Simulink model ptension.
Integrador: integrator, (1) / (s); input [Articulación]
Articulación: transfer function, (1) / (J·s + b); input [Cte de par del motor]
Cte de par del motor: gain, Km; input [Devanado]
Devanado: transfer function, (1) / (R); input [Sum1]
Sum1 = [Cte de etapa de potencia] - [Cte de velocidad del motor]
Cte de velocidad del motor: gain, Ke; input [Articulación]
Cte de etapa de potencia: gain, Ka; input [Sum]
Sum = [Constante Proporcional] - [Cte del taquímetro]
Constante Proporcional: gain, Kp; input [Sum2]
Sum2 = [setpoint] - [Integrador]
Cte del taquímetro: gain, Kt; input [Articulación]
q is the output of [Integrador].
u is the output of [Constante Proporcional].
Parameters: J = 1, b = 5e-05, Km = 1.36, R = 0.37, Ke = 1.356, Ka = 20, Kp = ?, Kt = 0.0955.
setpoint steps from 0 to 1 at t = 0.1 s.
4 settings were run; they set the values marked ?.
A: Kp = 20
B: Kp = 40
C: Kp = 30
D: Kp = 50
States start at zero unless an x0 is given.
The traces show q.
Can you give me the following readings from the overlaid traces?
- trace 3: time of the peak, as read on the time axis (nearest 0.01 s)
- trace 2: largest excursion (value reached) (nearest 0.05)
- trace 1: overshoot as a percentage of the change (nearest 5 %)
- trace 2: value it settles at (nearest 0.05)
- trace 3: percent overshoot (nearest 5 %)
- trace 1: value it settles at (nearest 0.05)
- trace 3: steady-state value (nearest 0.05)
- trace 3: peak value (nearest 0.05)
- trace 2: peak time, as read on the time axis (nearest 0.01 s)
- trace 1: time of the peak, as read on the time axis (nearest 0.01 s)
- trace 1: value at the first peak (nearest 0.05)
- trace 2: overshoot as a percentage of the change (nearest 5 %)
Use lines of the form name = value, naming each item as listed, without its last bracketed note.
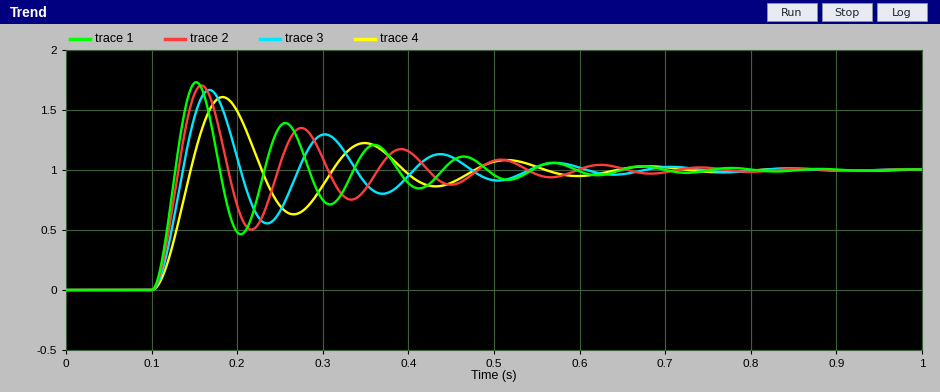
trace 3: time of the peak, as read on the time axis = 0.17 s
trace 2: largest excursion (value reached) = 1.70
trace 1: overshoot as a percentage of the change = 75 %
trace 2: value it settles at = 1.00
trace 3: percent overshoot = 65 %
trace 1: value it settles at = 1.00
trace 3: steady-state value = 1.00
trace 3: peak value = 1.65
trace 2: peak time, as read on the time axis = 0.16 s
trace 1: time of the peak, as read on the time axis = 0.15 s
trace 1: value at the first peak = 1.75
trace 2: overshoot as a percentage of the change = 70 %
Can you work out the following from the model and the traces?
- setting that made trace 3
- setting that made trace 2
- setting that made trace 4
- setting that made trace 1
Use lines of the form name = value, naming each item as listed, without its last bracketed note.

setting that made trace 3 = C
setting that made trace 2 = B
setting that made trace 4 = A
setting that made trace 1 = D
